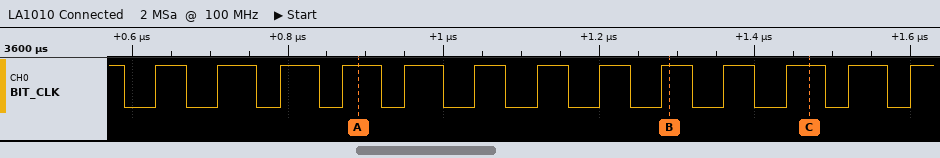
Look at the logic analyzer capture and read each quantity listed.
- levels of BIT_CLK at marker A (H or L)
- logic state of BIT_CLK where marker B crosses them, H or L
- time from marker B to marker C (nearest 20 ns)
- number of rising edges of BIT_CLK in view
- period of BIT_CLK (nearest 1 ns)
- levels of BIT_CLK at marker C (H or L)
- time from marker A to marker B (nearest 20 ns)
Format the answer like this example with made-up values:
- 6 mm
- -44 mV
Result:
- BIT_CLK=H
- BIT_CLK=H
- 180 ns
- 13
- 81 ns
- BIT_CLK=H
- 400 ns
